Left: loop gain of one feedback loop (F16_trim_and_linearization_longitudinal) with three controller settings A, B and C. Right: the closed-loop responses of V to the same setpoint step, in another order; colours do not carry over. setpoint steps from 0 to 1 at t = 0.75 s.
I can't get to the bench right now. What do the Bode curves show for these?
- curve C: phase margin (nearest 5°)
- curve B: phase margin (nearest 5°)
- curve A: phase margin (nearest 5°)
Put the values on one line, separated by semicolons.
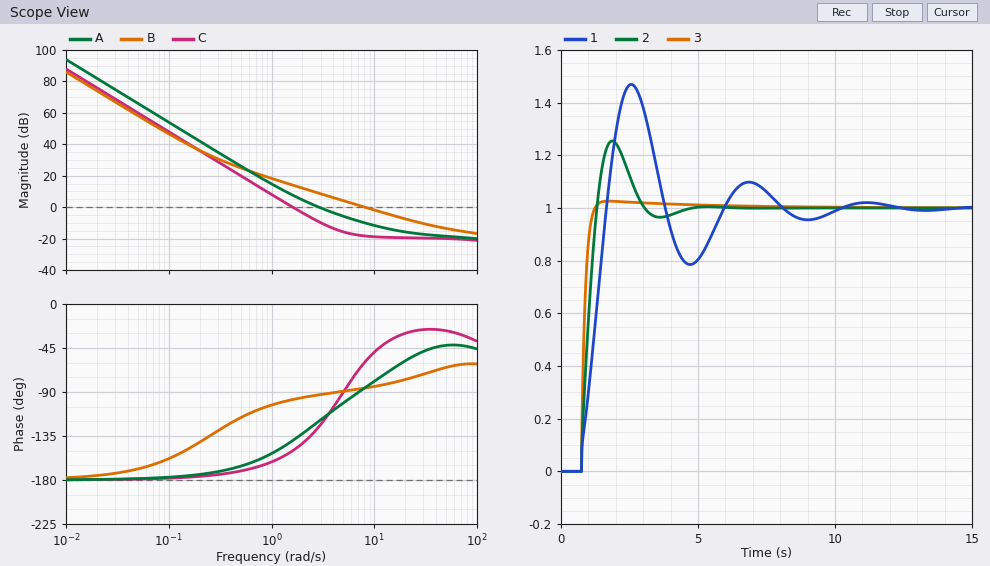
30°; 95°; 60°
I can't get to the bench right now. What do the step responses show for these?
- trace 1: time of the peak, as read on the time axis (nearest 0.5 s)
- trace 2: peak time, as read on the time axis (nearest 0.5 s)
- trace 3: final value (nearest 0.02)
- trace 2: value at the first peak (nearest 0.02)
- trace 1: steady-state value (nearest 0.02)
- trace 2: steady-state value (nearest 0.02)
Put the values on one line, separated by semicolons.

2.5 s; 2.0 s; 1.00; 1.26; 1.00; 1.00
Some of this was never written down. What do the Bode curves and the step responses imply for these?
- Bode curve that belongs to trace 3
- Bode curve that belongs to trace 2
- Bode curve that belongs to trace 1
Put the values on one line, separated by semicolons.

B; A; C
